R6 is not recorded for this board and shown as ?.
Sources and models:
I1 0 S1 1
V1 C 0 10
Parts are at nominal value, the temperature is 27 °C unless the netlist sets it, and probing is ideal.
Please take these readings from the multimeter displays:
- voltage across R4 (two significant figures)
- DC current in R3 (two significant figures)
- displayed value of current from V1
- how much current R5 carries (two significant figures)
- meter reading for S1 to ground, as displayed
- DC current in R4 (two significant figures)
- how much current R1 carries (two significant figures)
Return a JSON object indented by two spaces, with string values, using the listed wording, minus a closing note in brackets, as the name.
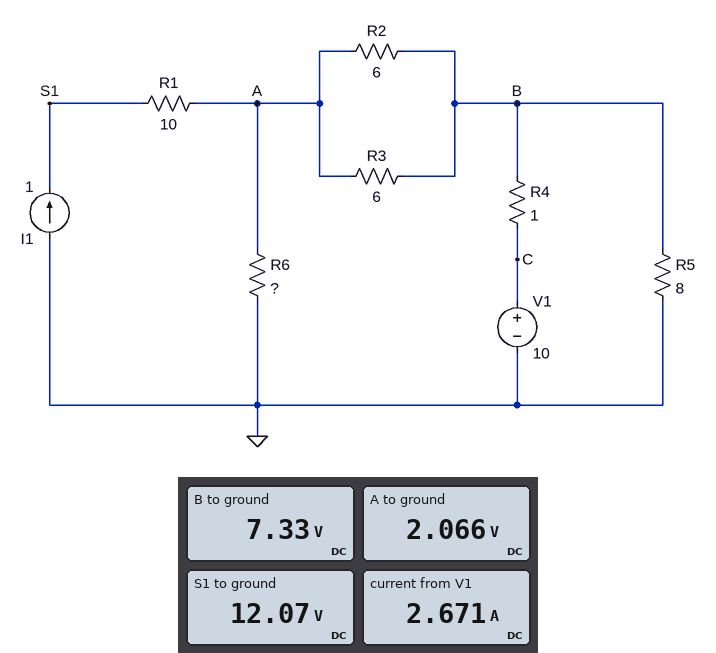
{
  "voltage across R4": "2.7 V",
  "DC current in R3": "880 mA",
  "displayed value of current from V1": "2.671 A",
  "how much current R5 carries": "920 mA",
  "meter reading for S1 to ground, as displayed": "12.07 V",
  "DC current in R4": "2.7 A",
  "how much current R1 carries": "1.0 A"
}
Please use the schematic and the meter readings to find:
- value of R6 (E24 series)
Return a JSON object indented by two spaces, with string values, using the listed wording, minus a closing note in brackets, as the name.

{
  "value of R6": "0.75 Ω"
}
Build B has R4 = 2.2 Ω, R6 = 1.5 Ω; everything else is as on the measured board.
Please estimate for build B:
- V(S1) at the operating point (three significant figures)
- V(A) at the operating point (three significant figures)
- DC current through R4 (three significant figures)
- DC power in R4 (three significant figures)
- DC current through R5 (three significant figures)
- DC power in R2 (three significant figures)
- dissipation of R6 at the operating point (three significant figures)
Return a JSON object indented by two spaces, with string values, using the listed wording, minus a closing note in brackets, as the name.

{
  "V(S1) at the operating point": "13.0 V",
  "V(A) at the operating point": "3.03 V",
  "DC current through R4": "1.78 A",
  "DC power in R4": "6.97 W",
  "DC current through R5": "761 mA",
  "DC power in R2": "1.56 W",
  "dissipation of R6 at the operating point": "6.11 W"
}
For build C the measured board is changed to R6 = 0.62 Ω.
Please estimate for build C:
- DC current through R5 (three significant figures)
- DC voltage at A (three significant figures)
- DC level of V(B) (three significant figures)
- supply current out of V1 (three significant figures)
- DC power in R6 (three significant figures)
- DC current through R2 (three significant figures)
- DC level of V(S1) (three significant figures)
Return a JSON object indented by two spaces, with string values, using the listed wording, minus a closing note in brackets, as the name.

{
  "DC current through R5": "907 mA",
  "DC voltage at A": "1.76 V",
  "DC level of V(B)": "7.26 V",
  "supply current out of V1": "2.74 A",
  "DC power in R6": "4.98 W",
  "DC current through R2": "917 mA",
  "DC level of V(S1)": "11.8 V"
}
